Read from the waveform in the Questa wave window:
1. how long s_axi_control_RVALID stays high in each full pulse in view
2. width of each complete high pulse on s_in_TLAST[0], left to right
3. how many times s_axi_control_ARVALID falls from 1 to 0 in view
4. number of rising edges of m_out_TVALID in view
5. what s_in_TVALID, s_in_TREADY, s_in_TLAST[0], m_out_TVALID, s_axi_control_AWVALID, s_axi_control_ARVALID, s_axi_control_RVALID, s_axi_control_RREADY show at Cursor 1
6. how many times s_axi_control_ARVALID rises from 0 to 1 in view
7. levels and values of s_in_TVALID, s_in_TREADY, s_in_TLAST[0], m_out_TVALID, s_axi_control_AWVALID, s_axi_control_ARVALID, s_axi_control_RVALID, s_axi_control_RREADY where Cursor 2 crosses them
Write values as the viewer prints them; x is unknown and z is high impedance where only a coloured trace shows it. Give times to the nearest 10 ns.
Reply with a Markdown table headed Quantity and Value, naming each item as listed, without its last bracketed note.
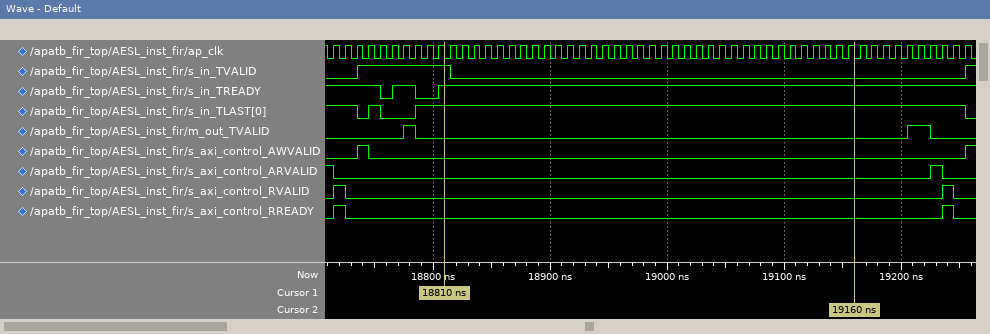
| Quantity | Value |
|---|---|
| how long s_axi_control_RVALID stays high in each full pulse in view | 10 ns, 10 ns |
| width of each complete high pulse on s_in_TLAST[0], left to right | 10 ns, 470 ns |
| how many times s_axi_control_ARVALID falls from 1 to 0 in view | 2 |
| number of rising edges of m_out_TVALID in view | 2 |
| what s_in_TVALID, s_in_TREADY, s_in_TLAST[0], m_out_TVALID, s_axi_control_AWVALID, s_axi_control_ARVALID, s_axi_control_RVALID, s_axi_control_RREADY show at Cursor 1 | s_in_TVALID=1, s_in_TREADY=1, s_in_TLAST[0]=1, m_out_TVALID=0, s_axi_control_AWVALID=0, s_axi_control_ARVALID=0, s_axi_control_RVALID=0, s_axi_control_RREADY=0 |
| how many times s_axi_control_ARVALID rises from 0 to 1 in view | 1 |
| levels and values of s_in_TVALID, s_in_TREADY, s_in_TLAST[0], m_out_TVALID, s_axi_control_AWVALID, s_axi_control_ARVALID, s_axi_control_RVALID, s_axi_control_RREADY where Cursor 2 crosses them | s_in_TVALID=0, s_in_TREADY=1, s_in_TLAST[0]=1, m_out_TVALID=0, s_axi_control_AWVALID=0, s_axi_control_ARVALID=0, s_axi_control_RVALID=0, s_axi_control_RREADY=0 |
